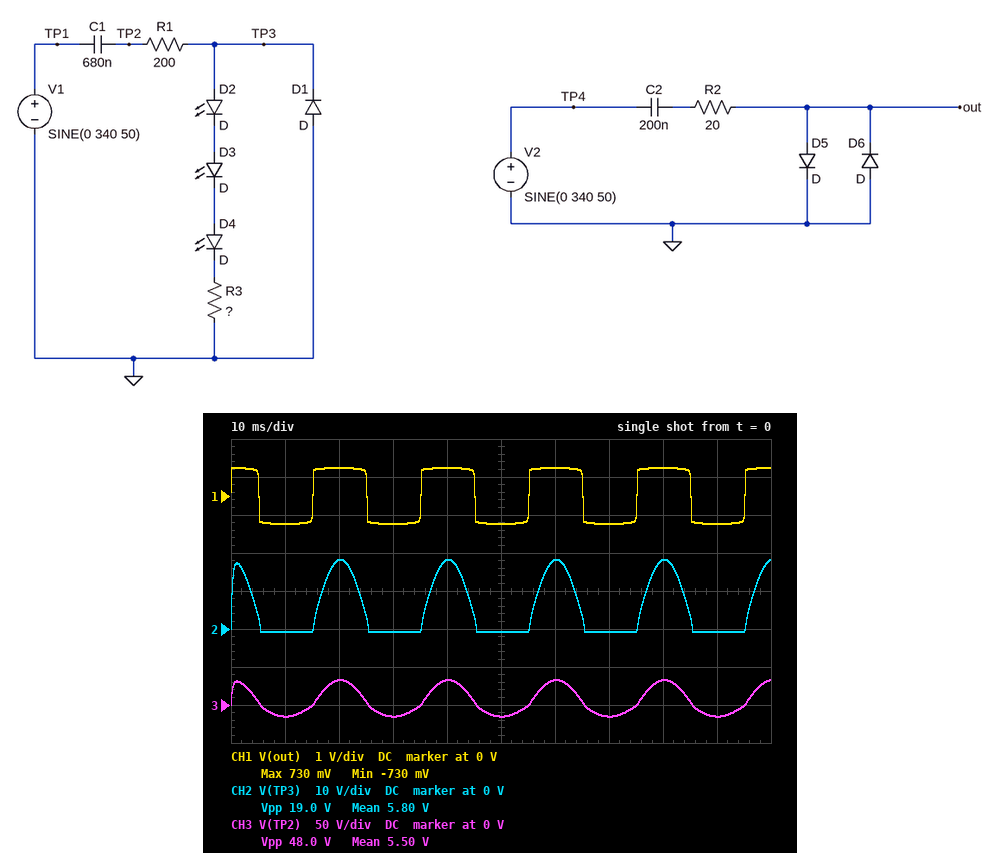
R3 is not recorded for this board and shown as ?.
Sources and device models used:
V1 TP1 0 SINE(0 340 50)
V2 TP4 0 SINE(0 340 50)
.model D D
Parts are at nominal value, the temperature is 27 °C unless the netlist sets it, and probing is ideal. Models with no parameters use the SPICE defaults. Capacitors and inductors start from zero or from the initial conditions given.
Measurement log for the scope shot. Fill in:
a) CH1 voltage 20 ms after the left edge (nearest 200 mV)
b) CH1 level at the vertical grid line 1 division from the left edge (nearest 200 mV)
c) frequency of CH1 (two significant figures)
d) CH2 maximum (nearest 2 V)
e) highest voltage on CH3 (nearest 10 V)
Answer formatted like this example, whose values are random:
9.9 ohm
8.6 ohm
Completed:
800 mV
-800 mV
50 Hz
18 V
30 V
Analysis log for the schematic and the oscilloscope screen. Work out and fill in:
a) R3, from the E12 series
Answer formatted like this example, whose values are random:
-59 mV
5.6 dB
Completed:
220 Ω
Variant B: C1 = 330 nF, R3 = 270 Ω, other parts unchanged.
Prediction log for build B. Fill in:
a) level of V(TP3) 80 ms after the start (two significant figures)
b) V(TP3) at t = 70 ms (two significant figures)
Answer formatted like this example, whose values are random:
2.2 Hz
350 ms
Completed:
12 V
-750 mV
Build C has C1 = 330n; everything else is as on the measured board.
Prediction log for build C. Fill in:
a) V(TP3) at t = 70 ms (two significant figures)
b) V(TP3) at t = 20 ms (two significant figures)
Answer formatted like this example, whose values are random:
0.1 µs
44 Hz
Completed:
-750 mV
10 V
